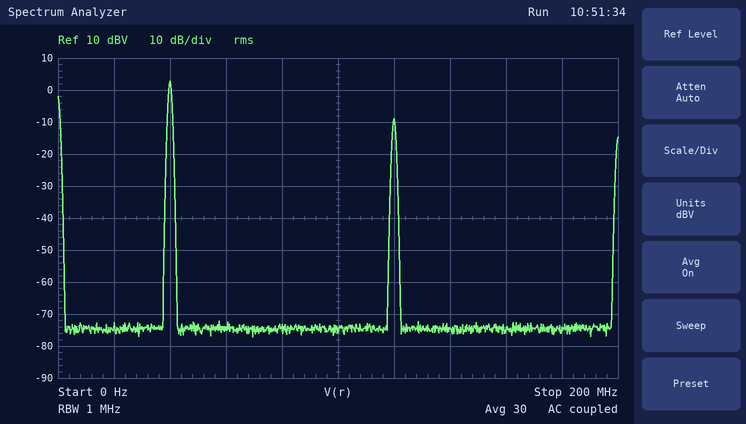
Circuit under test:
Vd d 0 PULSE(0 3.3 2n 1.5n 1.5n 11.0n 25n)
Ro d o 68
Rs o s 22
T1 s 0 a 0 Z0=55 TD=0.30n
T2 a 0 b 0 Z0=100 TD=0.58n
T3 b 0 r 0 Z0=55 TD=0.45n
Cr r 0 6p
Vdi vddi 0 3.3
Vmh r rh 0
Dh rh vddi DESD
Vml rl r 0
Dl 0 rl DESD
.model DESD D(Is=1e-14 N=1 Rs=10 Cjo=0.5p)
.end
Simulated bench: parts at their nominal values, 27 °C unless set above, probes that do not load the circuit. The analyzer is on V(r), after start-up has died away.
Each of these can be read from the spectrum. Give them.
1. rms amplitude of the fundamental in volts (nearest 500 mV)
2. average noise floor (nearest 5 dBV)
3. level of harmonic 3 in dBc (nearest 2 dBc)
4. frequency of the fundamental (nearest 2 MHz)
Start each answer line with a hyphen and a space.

- 1.5 V
- -75 dBV
- -12 dBc
- 40 MHz
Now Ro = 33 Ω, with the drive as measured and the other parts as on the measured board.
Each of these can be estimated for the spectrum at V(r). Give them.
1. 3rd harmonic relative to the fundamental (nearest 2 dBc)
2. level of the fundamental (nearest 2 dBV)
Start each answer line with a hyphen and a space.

- -8 dBc
- 4 dBV
